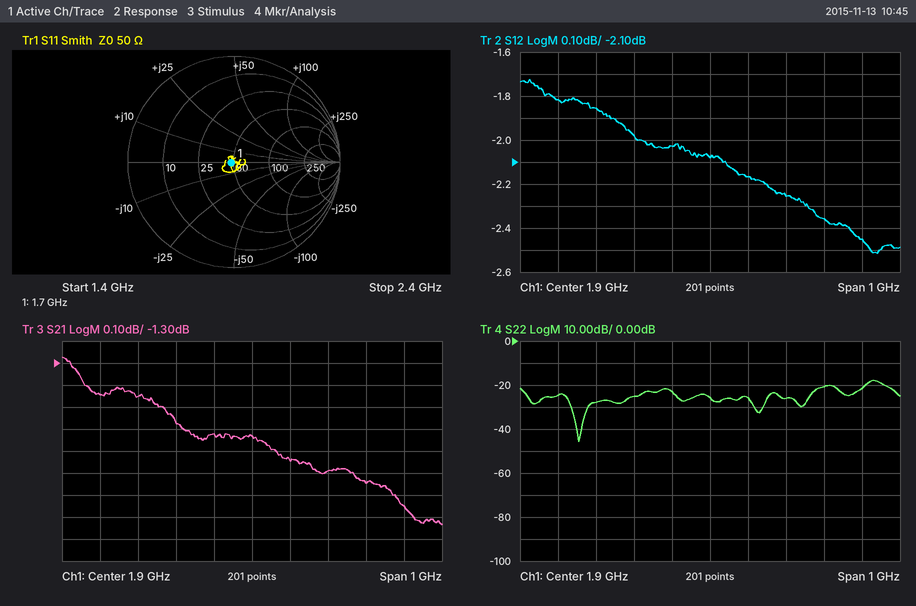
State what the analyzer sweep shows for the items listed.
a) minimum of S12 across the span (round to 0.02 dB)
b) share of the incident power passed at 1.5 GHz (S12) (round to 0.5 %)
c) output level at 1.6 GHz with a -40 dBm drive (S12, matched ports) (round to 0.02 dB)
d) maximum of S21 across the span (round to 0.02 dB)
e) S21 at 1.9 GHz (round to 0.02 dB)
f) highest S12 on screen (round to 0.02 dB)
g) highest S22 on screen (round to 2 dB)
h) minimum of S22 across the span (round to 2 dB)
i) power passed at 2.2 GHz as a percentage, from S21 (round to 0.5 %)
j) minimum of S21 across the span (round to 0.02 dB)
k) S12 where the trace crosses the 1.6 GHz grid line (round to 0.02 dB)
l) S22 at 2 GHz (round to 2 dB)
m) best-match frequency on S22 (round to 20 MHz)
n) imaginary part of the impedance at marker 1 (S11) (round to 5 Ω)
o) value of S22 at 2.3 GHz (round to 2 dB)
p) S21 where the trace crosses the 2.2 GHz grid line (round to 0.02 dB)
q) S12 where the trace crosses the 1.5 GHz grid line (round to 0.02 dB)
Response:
-2.52 dB
66.0 %
-41.86 dBm
-1.28 dB
-1.64 dB
-1.72 dB
-18 dB
-46 dB
65.5 %
-2.04 dB
-1.86 dB
-26 dB
1.56 GHz
0 Ω
-22 dB
-1.84 dB
-1.82 dB
